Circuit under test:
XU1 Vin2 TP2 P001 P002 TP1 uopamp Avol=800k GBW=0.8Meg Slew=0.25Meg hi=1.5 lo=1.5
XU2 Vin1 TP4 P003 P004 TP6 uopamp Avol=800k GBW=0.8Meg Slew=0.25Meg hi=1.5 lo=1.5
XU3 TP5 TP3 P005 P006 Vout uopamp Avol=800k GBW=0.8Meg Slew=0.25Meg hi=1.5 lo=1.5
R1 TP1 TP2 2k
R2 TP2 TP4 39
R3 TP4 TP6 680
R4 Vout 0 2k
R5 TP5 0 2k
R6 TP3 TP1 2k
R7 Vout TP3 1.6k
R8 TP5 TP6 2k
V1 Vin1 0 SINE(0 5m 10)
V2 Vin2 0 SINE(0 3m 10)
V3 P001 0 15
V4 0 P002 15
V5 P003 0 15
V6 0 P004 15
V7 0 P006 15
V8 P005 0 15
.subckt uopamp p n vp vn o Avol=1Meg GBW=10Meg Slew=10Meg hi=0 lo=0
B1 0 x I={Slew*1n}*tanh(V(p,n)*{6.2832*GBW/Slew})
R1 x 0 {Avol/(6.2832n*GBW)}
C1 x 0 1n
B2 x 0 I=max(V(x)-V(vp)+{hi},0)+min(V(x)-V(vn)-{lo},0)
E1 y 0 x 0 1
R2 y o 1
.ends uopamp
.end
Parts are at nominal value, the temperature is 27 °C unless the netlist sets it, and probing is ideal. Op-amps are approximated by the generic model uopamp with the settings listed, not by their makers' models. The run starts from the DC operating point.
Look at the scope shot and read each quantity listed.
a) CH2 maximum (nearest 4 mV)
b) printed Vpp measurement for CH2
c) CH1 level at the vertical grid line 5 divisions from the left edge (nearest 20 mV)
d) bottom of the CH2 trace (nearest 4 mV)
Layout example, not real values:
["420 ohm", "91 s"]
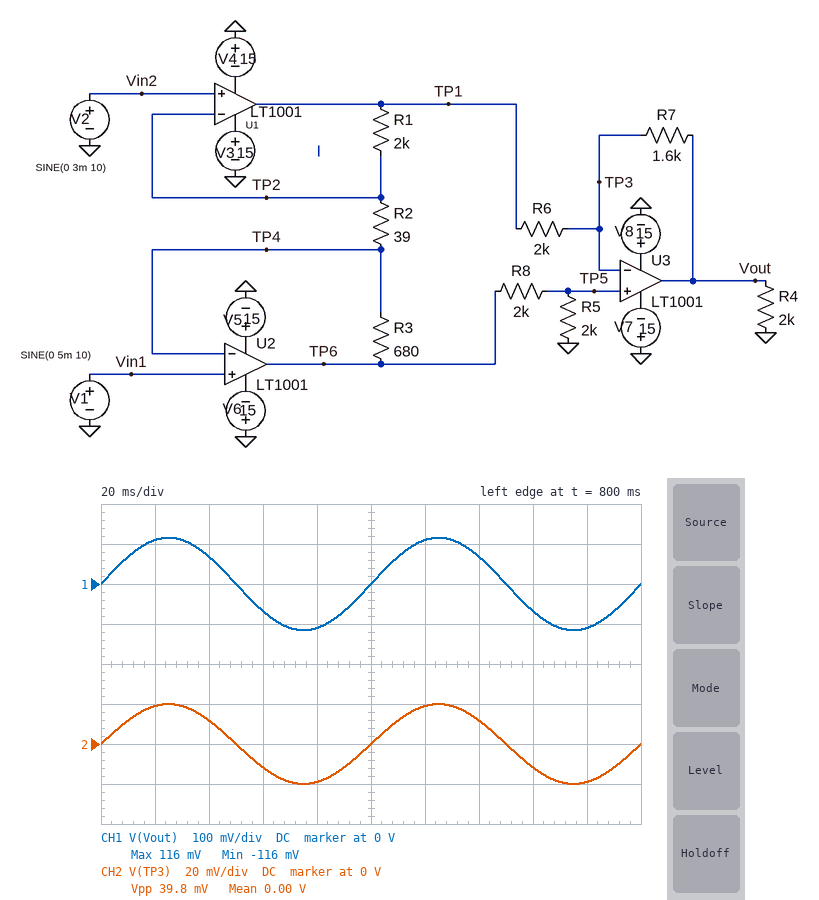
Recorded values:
["20 mV", "39.8 mV", "0 V", "-20 mV"]
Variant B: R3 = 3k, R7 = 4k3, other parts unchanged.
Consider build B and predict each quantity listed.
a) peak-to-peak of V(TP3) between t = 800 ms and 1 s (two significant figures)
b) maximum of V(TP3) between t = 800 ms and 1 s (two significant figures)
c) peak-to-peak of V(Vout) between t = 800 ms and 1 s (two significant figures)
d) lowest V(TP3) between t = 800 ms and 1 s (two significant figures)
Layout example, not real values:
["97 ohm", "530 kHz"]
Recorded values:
["160 mV", "79 mV", "930 mV", "-79 mV"]
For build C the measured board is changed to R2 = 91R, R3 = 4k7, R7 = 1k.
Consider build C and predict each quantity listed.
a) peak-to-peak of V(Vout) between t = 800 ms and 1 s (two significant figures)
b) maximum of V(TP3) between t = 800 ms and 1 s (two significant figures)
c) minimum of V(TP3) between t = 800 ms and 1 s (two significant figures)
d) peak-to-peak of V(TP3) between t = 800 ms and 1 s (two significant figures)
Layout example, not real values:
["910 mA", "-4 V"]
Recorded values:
["200 mV", "54 mV", "-54 mV", "110 mV"]
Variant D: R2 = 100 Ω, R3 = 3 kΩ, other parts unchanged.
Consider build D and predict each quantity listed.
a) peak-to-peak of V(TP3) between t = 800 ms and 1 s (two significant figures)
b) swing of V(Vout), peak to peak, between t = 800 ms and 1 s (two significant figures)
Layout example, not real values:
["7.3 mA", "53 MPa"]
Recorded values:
["65 mV", "180 mV"]
